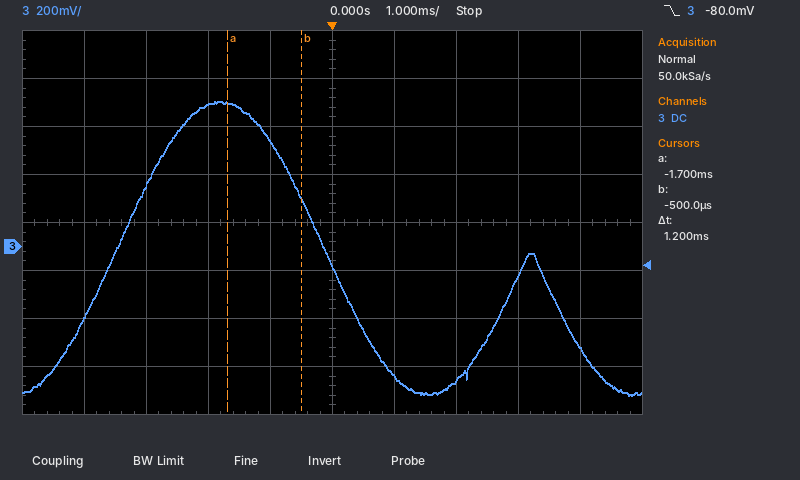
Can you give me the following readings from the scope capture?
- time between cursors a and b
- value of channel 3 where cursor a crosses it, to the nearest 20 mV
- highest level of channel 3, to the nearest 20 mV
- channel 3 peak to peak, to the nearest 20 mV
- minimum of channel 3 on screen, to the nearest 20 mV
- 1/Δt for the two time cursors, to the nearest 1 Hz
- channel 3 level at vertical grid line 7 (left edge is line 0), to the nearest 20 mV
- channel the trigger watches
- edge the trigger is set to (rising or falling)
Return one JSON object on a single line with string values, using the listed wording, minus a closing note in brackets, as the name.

{"time between cursors a and b": "1.2 ms", "value of channel 3 where cursor a crosses it, to the nearest 20 mV": "600 mV", "highest level of channel 3, to the nearest 20 mV": "600 mV", "channel 3 peak to peak, to the nearest 20 mV": "1.22 V", "minimum of channel 3 on screen, to the nearest 20 mV": "-620 mV", "1/Δt for the two time cursors, to the nearest 1 Hz": "833 Hz", "channel 3 level at vertical grid line 7 (left edge is line 0), to the nearest 20 mV": "-560 mV", "channel the trigger watches": "channel 3", "edge the trigger is set to": "falling"}
